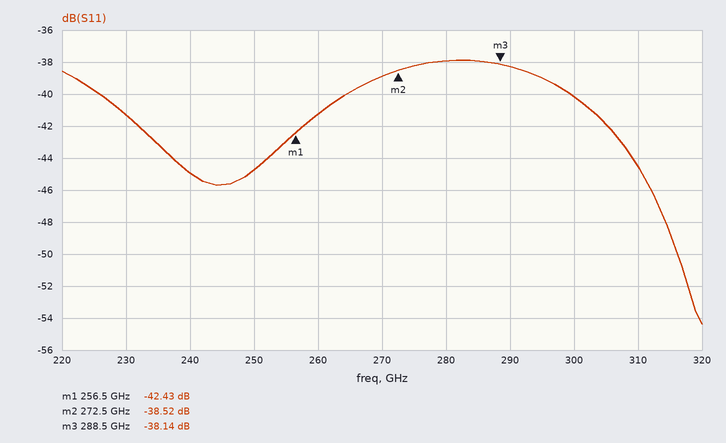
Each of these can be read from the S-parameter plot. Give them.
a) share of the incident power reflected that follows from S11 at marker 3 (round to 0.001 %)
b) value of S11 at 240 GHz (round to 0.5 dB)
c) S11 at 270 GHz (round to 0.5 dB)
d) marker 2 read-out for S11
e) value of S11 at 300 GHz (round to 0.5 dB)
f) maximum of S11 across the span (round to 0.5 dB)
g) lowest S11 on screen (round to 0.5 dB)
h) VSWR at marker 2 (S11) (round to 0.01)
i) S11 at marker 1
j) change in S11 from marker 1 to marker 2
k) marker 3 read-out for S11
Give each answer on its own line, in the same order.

0.015 %
-45.0 dB
-39.0 dB
-38.52 dB
-40.0 dB
-38.0 dB
-54.5 dB
1.02
-42.43 dB
3.91 dB
-38.14 dB
